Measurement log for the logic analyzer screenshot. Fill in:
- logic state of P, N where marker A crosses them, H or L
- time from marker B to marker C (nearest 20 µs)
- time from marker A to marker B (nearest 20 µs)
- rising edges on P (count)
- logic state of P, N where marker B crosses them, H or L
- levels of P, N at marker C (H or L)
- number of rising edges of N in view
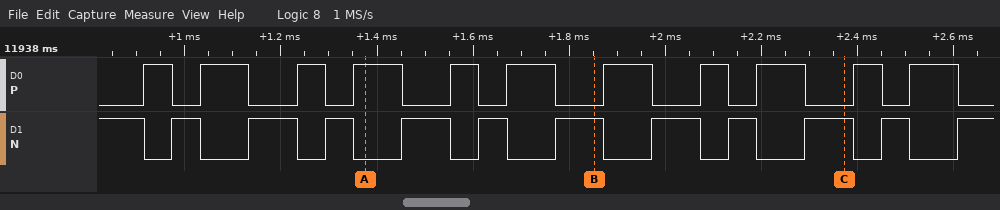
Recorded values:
P=H, N=L
520 µs
480 µs
11
P=L, N=H
P=L, N=H
11
